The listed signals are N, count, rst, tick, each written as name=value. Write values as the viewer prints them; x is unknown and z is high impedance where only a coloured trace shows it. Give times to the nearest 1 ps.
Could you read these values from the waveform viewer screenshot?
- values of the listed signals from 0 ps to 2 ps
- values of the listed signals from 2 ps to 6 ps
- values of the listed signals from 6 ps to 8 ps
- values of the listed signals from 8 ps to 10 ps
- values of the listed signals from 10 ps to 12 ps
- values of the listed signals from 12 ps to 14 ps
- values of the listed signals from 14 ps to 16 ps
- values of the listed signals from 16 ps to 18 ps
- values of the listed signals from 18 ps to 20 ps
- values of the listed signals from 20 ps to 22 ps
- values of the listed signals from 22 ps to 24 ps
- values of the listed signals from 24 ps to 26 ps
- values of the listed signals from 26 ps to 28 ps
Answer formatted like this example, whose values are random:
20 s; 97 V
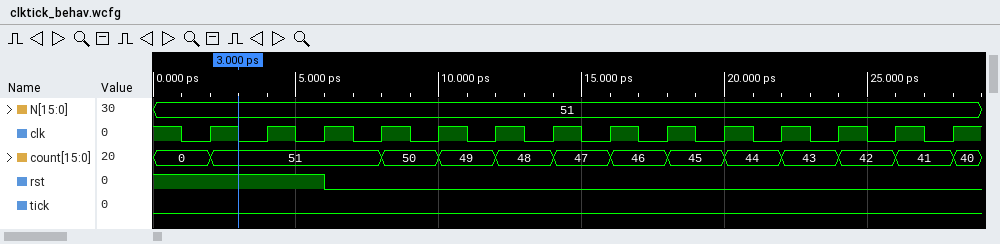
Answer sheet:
N=51, count=0, rst=1, tick=0; N=51, count=51, rst=1, tick=0; N=51, count=51, rst=0, tick=0; N=51, count=50, rst=0, tick=0; N=51, count=49, rst=0, tick=0; N=51, count=48, rst=0, tick=0; N=51, count=47, rst=0, tick=0; N=51, count=46, rst=0, tick=0; N=51, count=45, rst=0, tick=0; N=51, count=44, rst=0, tick=0; N=51, count=43, rst=0, tick=0; N=51, count=42, rst=0, tick=0; N=51, count=41, rst=0, tick=0
